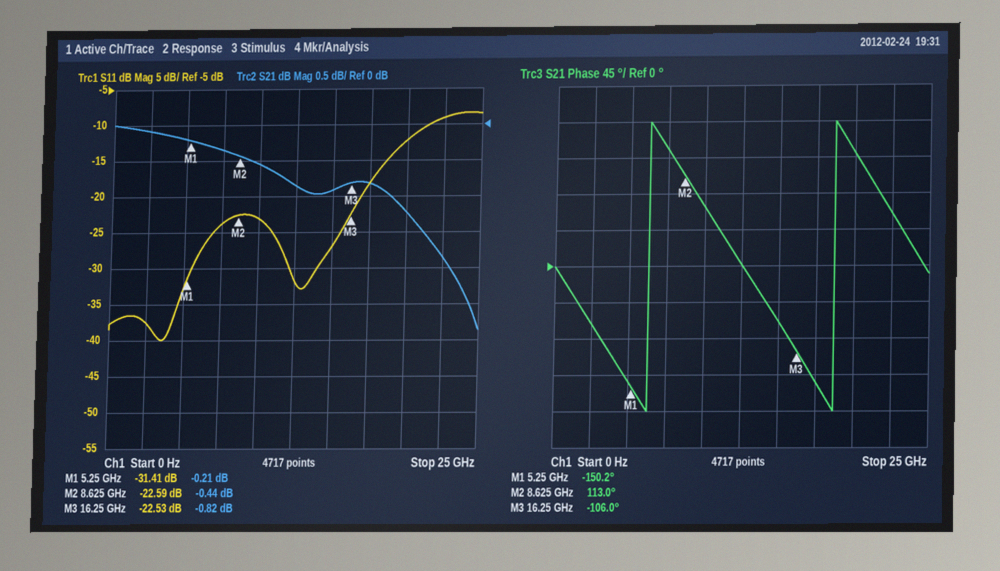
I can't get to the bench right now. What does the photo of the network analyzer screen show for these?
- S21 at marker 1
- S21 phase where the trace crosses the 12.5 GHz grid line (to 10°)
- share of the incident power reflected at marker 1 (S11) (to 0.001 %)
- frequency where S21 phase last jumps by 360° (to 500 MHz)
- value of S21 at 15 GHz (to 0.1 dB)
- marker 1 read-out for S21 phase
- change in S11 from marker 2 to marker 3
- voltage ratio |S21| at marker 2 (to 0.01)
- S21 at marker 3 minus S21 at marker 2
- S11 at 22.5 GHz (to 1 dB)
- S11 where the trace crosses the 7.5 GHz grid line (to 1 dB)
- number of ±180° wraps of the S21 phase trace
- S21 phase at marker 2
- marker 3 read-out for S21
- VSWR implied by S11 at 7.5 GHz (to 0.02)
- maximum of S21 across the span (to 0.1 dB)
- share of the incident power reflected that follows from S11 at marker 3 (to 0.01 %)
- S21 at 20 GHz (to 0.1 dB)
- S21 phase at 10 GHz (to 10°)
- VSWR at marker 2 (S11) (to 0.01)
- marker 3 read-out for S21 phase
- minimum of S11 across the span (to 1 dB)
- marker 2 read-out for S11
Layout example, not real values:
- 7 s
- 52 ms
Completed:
- -0.21 dB
- 0°
- 0.072 %
- 18.5 GHz
- -0.9 dB
- -150.2°
- 0.06 dB
- 0.95
- -0.38 dB
- -9 dB
- -24 dB
- 2
- 113.0°
- -0.82 dB
- 1.14
- 0.0 dB
- 0.56 %
- -1.2 dB
- 70°
- 1.16
- -106.0°
- -40 dB
- -22.59 dB
